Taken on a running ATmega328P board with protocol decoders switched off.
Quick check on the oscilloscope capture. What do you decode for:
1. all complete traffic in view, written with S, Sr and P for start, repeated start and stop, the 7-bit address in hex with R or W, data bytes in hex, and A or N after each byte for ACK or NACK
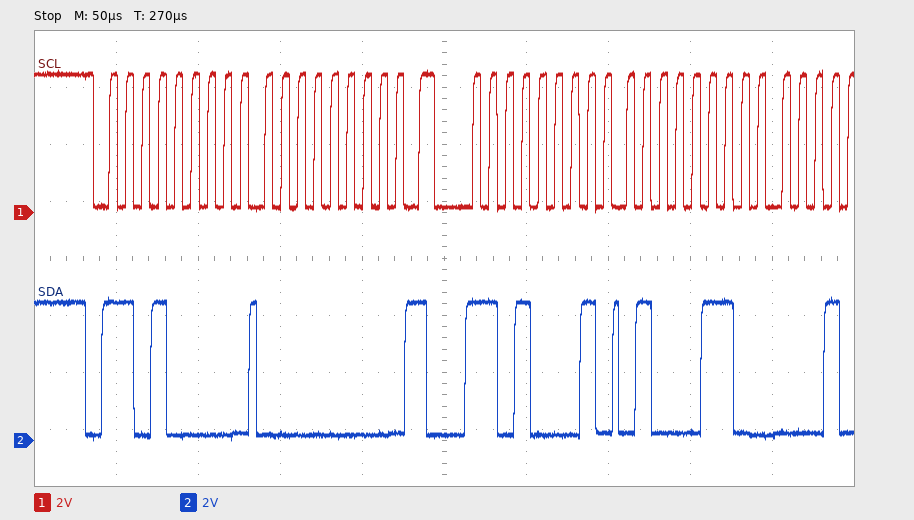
S 68W A 00 A Sr 68R A 46 A
